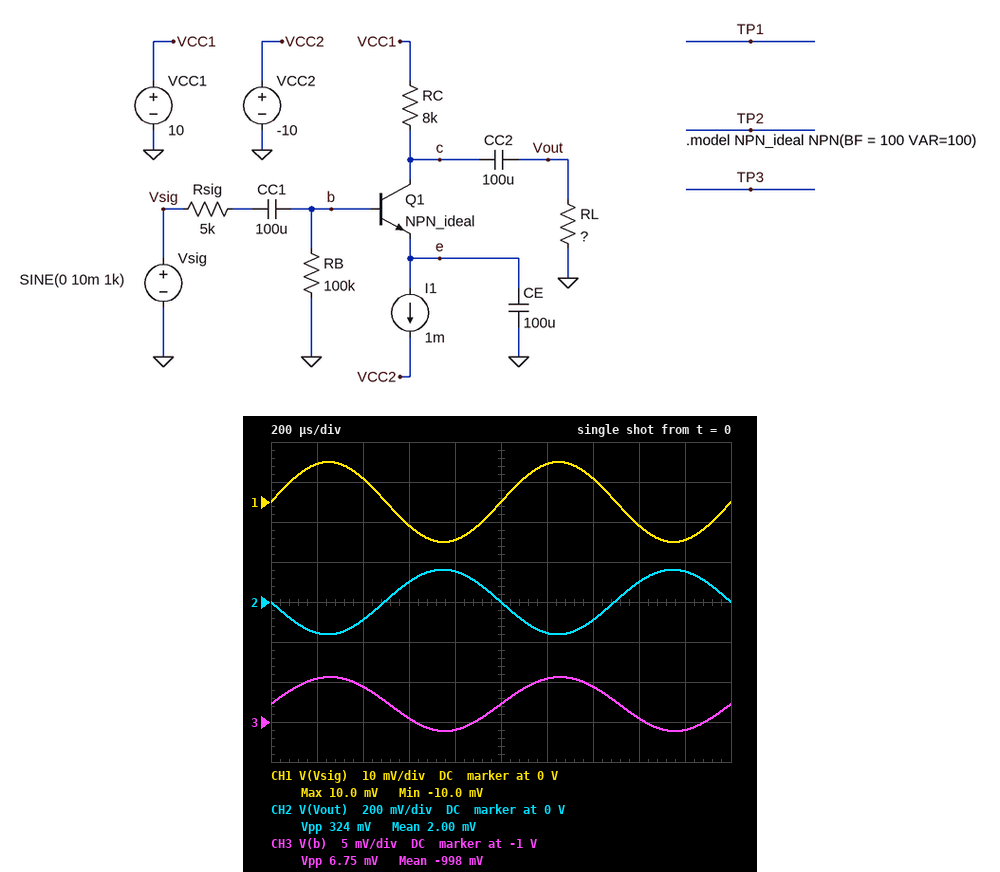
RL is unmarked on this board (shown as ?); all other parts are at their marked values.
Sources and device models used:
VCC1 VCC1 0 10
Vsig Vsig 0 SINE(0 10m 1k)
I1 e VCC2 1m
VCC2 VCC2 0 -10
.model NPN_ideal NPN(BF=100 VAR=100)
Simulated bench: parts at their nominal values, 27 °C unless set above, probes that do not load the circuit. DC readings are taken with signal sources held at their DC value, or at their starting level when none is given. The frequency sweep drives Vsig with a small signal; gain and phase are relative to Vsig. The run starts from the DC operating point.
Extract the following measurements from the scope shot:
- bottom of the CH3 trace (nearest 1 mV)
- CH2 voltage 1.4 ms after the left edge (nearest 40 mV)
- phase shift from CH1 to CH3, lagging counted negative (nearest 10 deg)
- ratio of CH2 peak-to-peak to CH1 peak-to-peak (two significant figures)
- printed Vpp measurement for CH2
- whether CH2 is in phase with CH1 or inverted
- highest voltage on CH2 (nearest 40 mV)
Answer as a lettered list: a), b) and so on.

a) -1.001 V
b) -80 mV
c) 0 deg
d) 16
e) 324 mV
f) inverted
g) 160 mV
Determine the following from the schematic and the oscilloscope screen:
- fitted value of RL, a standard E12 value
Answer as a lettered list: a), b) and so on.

a) 1.5 kΩ
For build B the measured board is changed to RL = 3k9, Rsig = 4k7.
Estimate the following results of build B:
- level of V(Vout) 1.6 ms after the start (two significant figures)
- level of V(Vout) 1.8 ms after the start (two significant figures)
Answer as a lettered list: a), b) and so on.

a) 220 mV
b) 330 mV
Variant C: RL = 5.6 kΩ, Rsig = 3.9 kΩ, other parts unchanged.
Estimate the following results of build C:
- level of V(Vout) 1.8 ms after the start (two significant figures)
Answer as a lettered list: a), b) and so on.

a) 460 mV
